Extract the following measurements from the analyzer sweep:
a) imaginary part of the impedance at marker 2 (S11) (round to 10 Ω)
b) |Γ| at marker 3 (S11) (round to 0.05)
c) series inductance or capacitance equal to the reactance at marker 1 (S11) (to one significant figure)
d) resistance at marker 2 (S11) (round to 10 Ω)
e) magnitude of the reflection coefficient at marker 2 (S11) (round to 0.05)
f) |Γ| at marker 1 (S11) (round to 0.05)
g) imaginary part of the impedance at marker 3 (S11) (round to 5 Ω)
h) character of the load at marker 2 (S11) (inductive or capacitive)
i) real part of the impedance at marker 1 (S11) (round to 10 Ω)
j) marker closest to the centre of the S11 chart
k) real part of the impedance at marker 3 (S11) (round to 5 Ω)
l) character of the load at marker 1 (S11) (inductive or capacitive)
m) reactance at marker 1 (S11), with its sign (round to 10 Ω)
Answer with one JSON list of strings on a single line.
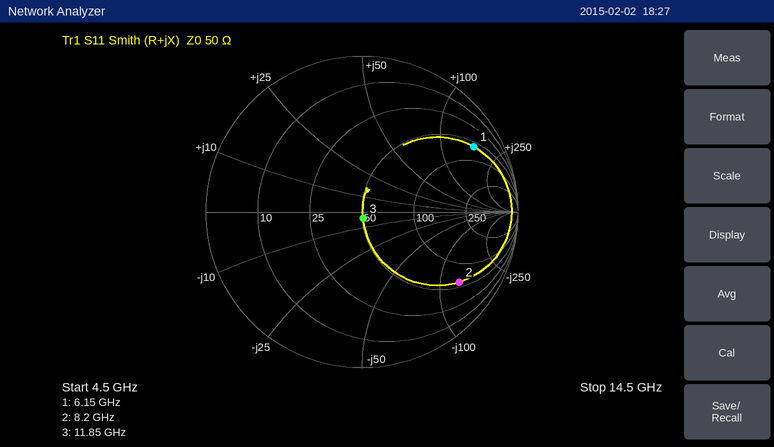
["-130 Ω", "0.05", "4 nH", "60 Ω", "0.75", "0.85", "-5 Ω", "capacitive", "60 Ω", "marker 3", "50 Ω", "inductive", "+160 Ω"]
